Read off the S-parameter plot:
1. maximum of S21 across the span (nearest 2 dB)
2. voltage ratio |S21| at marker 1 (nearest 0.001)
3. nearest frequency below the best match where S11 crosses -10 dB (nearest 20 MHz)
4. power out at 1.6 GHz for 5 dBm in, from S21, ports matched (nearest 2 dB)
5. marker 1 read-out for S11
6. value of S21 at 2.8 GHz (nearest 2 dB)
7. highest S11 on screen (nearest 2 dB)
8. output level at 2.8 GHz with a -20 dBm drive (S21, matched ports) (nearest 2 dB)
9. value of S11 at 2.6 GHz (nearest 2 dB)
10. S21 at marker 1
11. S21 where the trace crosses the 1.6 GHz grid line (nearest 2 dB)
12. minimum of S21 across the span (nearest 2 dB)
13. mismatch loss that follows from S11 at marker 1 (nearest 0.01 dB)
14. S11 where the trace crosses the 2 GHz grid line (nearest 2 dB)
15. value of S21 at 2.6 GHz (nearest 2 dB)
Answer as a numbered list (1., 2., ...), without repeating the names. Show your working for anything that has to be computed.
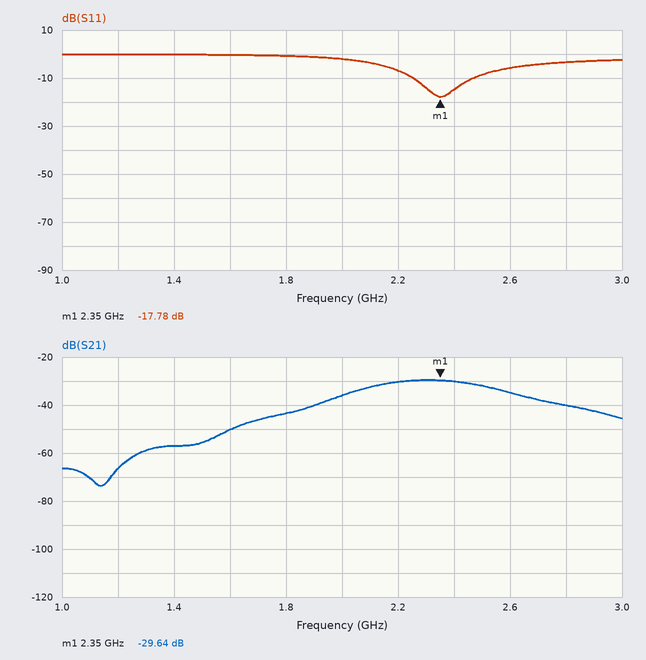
1. -30 dB
2. 10^(-29.64/20) ≈ 0.033
3. 2.26 GHz
4. 5 dBm + (-50 dB) = -46 dBm
5. -17.78 dB
6. -40 dB
7. 0 dB
8. -20 dBm + (-40 dB) = -60 dBm
9. -6 dB
10. -29.64 dB
11. -50 dB
12. -74 dB
13. −10 log10(1 − 10^(-17.78/10)) ≈ 0.07 dB
14. -2 dB
15. -34 dB
